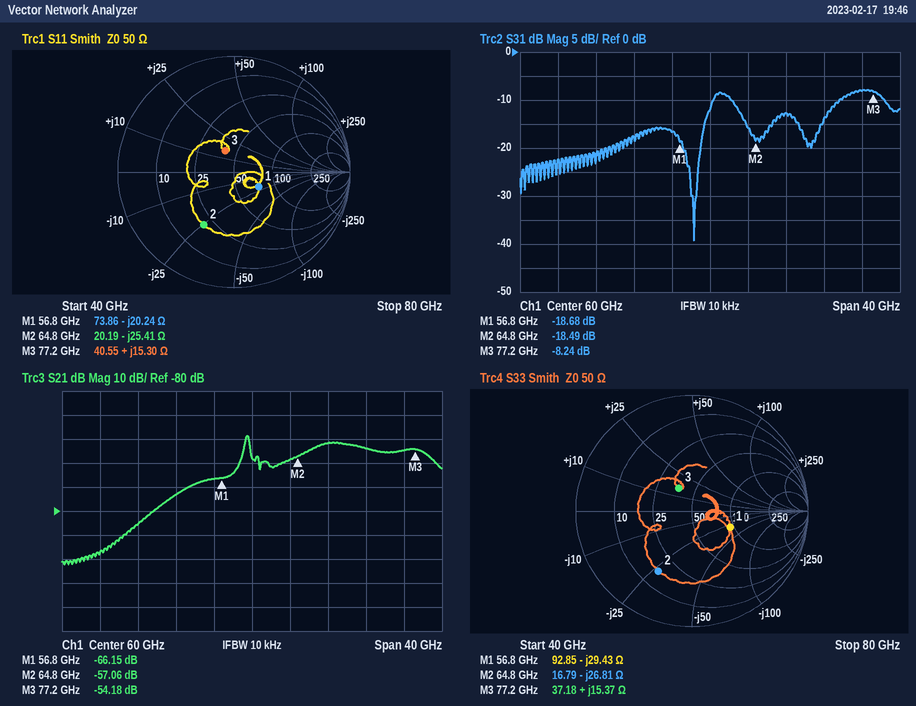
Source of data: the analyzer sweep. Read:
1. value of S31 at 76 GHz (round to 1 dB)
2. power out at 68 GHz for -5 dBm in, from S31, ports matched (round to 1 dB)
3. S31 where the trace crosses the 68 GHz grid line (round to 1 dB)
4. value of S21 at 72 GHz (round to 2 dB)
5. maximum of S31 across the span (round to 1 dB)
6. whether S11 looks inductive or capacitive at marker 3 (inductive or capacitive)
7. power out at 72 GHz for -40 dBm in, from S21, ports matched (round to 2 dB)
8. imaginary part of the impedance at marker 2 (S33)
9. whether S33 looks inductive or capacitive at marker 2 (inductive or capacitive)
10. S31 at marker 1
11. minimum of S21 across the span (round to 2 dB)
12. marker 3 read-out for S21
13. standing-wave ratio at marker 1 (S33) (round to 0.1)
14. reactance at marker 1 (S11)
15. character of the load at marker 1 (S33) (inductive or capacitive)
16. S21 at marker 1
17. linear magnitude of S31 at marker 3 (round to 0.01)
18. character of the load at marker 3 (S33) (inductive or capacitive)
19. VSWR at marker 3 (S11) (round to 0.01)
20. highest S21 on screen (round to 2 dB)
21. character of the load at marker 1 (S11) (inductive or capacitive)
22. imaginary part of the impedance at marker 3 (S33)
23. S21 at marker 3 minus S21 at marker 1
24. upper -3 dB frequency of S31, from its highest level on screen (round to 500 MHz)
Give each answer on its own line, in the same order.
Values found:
-8 dB
-18 dBm
-13 dB
-54 dB
-8 dB
inductive
-94 dBm
-26.81 Ω
capacitive
-18.68 dB
-102 dB
-54.18 dB
2.1
-20.24 Ω
capacitive
-66.15 dB
0.39
inductive
1.49
-48 dB
capacitive
+15.37 Ω
11.97 dB
78.5 GHz
